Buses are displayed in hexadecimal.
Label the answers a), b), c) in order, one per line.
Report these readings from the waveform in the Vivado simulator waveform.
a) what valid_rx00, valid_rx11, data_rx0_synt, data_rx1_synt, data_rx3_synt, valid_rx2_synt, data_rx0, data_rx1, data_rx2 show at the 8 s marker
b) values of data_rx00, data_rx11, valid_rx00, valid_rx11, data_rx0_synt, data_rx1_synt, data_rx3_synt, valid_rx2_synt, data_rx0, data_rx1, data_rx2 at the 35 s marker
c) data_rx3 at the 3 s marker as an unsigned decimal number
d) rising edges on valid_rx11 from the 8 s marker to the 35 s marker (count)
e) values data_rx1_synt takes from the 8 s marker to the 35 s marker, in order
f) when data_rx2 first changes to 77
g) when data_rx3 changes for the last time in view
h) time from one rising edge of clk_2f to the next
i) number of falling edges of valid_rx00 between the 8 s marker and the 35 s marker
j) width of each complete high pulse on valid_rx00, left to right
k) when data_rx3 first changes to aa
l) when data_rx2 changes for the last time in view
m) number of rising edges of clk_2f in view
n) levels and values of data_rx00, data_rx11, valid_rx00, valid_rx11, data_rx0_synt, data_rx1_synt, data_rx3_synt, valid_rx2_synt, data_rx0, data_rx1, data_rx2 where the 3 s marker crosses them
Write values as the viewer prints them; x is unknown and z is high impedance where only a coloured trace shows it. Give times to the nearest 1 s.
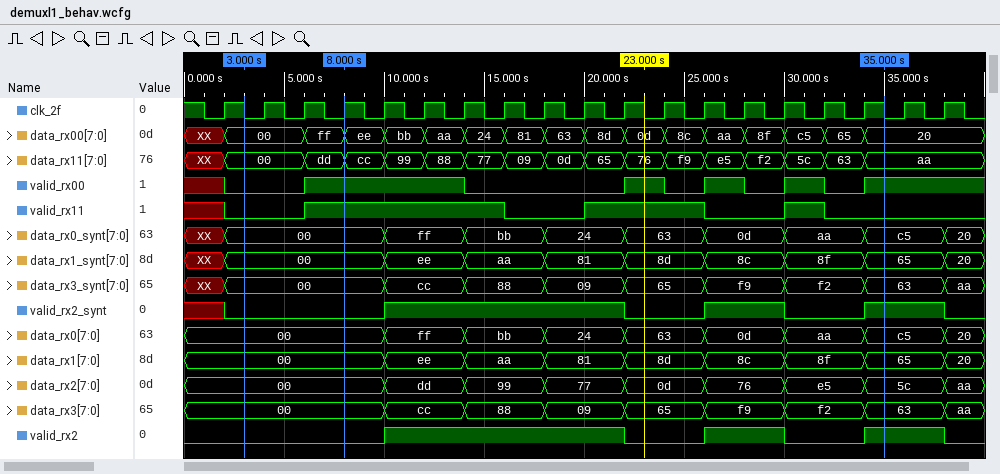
a) valid_rx00=1, valid_rx11=1, data_rx0_synt=00, data_rx1_synt=00, data_rx3_synt=00, valid_rx2_synt=0, data_rx0=00, data_rx1=00, data_rx2=00
b) data_rx00=20, data_rx11=aa, valid_rx00=1, valid_rx11=0, data_rx0_synt=c5, data_rx1_synt=65, data_rx3_synt=63, valid_rx2_synt=1, data_rx0=c5, data_rx1=65, data_rx2=5c
c) 0
d) 2
e) 00, ee, aa, 81, 8d, 8c, 8f, 65
f) 18 s
g) 38 s
h) 2 s
i) 4
j) 8 s, 2 s, 2 s, 2 s
k) 38 s
l) 38 s
m) 19
n) data_rx00=00, data_rx11=00, valid_rx00=0, valid_rx11=0, data_rx0_synt=00, data_rx1_synt=00, data_rx3_synt=00, valid_rx2_synt=0, data_rx0=00, data_rx1=00, data_rx2=00
